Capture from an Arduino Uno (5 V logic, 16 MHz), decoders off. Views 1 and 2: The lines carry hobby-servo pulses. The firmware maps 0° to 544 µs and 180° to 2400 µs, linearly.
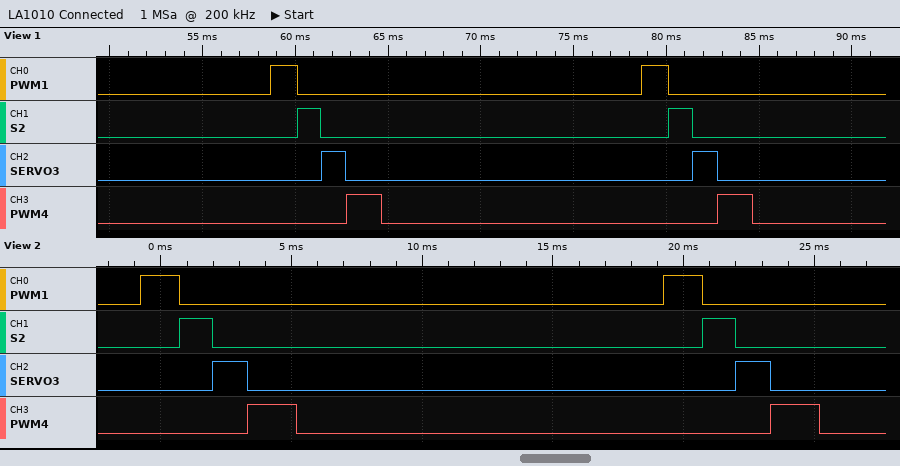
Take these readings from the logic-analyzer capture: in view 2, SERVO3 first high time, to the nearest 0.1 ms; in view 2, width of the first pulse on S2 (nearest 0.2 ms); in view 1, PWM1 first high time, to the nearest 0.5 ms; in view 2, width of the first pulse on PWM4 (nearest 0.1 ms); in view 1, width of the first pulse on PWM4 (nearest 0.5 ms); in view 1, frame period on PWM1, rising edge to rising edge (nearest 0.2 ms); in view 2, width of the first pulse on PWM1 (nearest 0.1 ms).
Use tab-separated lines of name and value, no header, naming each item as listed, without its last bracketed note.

in view 2, SERVO3 first high time, to the nearest 0.1 ms	1.3 ms
in view 2, width of the first pulse on S2	1.2 ms
in view 1, PWM1 first high time, to the nearest 0.5 ms	1.5 ms
in view 2, width of the first pulse on PWM4	1.9 ms
in view 1, width of the first pulse on PWM4	2.0 ms
in view 1, frame period on PWM1, rising edge to rising edge	20.0 ms
in view 2, width of the first pulse on PWM1	1.5 ms
